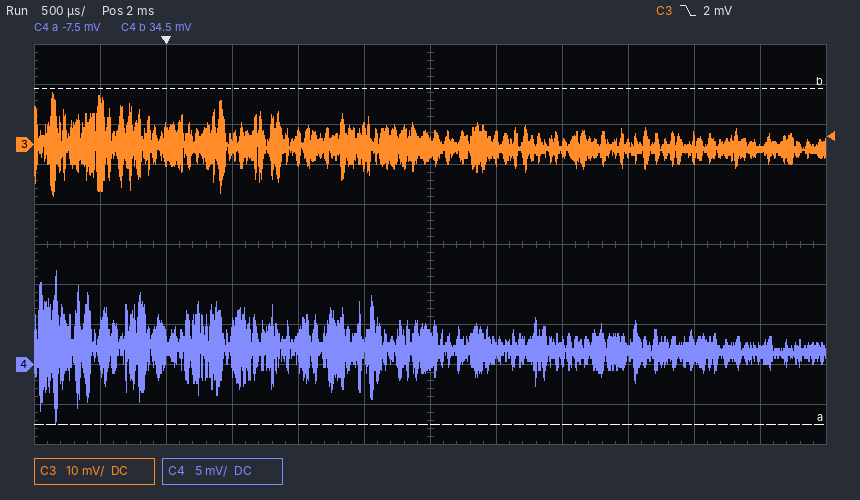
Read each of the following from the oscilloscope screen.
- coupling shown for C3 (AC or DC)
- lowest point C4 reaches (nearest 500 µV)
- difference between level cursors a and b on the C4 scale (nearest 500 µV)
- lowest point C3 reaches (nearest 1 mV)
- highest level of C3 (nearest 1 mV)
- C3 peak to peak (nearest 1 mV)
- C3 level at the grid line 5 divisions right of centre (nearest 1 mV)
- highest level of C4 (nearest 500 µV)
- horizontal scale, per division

DC
-7.5 mV
42.0 mV
-13 mV
13 mV
26 mV
-1 mV
12.0 mV
500 µs
